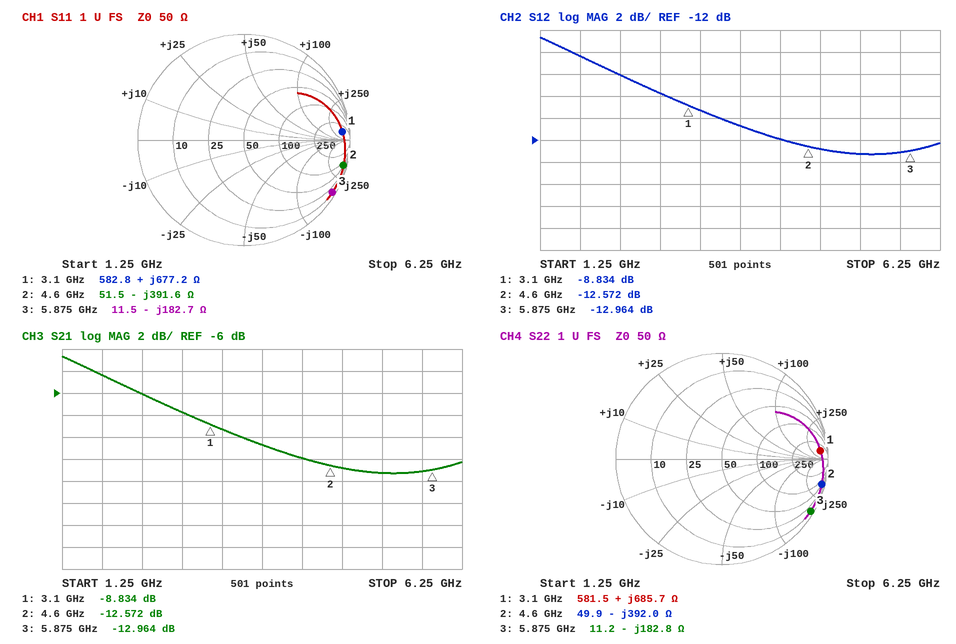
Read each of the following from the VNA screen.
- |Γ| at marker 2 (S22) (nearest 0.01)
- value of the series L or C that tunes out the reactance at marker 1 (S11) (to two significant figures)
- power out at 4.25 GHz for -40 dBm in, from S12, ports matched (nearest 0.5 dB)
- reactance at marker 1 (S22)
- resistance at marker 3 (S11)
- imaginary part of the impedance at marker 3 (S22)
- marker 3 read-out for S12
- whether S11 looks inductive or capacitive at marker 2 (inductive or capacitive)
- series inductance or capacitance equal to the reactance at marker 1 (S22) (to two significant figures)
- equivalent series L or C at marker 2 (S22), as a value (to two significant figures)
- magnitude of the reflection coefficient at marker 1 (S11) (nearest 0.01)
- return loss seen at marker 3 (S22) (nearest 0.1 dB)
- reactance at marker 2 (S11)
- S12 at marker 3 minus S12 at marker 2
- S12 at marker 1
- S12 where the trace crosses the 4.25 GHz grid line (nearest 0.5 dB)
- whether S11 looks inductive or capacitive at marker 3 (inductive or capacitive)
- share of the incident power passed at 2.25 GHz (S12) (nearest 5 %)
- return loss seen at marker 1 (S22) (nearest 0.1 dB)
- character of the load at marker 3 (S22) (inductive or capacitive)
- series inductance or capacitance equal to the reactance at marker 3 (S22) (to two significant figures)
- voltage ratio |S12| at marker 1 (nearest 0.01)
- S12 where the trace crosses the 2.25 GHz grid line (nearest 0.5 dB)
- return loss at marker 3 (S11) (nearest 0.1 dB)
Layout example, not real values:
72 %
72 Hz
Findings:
0.97
76 fF
-52.0 dBm
+685.7 Ω
11.5 Ω
-182.8 Ω
-12.964 dB
capacitive
35 nH
88 fF
0.93
0.3 dB
-391.6 Ω
-0.392 dB
-8.834 dB
-12.0 dB
capacitive
25 %
0.6 dB
capacitive
150 fF
0.36
-6.0 dB
0.3 dB
